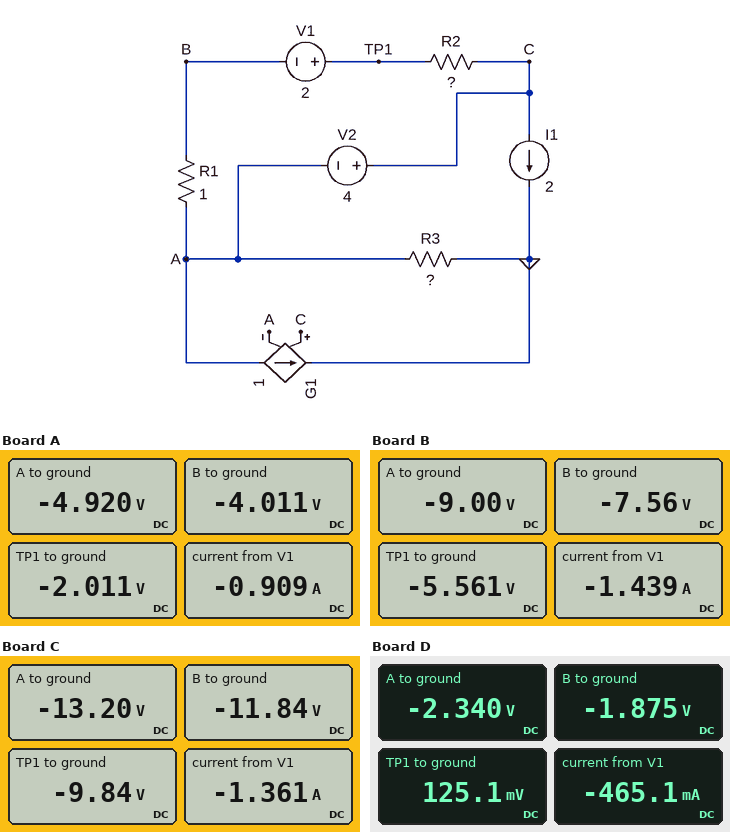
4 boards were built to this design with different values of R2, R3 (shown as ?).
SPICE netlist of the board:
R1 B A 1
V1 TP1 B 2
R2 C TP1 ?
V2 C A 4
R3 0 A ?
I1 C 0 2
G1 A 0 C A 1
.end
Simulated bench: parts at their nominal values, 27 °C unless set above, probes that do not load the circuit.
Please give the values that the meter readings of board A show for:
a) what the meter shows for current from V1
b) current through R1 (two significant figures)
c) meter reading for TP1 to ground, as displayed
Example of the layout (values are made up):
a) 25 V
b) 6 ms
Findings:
a) -0.909 A
b) 910 mA
c) -2.011 V
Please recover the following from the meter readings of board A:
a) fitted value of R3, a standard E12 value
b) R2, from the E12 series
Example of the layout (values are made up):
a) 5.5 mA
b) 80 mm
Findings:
a) 0.82 Ω
b) 1.2 Ω
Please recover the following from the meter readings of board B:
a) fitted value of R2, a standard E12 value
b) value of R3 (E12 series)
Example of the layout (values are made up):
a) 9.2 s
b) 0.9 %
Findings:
a) 0.39 Ω
b) 1.5 Ω
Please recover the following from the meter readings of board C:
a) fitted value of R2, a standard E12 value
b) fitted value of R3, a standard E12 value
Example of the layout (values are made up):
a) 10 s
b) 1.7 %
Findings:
a) 0.47 Ω
b) 2.2 Ω
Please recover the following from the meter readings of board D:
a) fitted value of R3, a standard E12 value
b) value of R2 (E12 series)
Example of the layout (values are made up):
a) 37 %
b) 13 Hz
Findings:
a) 0.39 Ω
b) 3.3 Ω
